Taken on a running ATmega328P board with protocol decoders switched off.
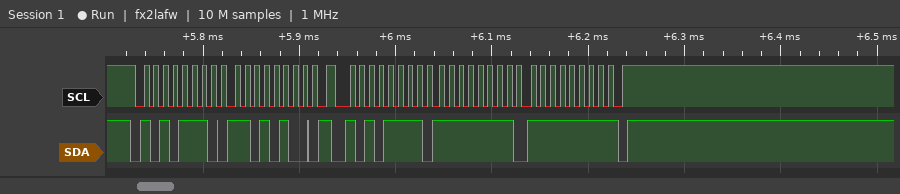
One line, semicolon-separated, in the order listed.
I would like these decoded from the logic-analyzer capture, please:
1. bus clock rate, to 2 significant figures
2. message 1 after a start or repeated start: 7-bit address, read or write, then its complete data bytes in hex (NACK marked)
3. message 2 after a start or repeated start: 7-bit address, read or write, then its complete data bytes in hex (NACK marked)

100 kHz; 0x57 write: D4; 0x57 read: FF FF NACK
